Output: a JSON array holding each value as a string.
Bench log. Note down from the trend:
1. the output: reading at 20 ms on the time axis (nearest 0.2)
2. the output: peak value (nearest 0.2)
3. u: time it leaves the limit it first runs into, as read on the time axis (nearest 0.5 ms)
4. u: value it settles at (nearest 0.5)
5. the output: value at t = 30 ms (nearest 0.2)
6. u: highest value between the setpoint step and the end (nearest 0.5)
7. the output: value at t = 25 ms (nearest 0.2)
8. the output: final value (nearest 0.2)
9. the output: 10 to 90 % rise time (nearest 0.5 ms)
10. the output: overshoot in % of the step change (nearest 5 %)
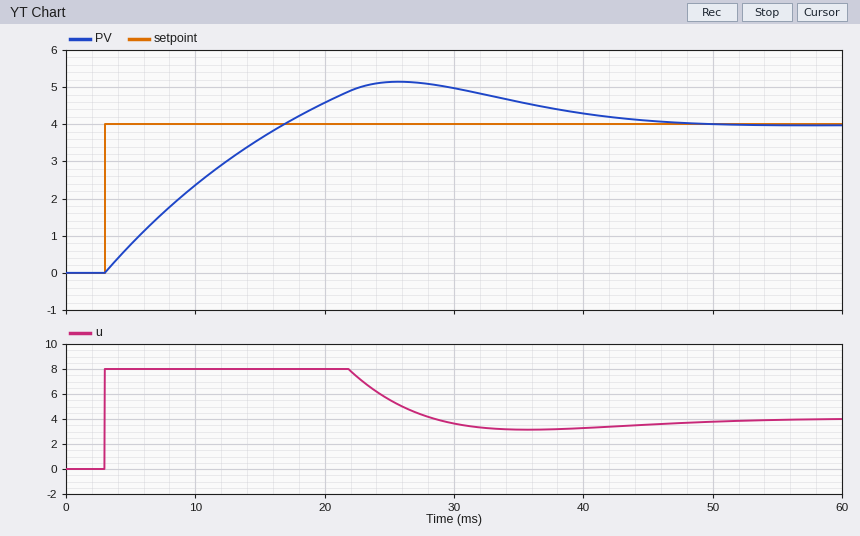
["4.6", "5.2", "22.0 ms", "4.0", "5.0", "8.0", "5.2", "4.0", "11.0 ms", "30 %"]
